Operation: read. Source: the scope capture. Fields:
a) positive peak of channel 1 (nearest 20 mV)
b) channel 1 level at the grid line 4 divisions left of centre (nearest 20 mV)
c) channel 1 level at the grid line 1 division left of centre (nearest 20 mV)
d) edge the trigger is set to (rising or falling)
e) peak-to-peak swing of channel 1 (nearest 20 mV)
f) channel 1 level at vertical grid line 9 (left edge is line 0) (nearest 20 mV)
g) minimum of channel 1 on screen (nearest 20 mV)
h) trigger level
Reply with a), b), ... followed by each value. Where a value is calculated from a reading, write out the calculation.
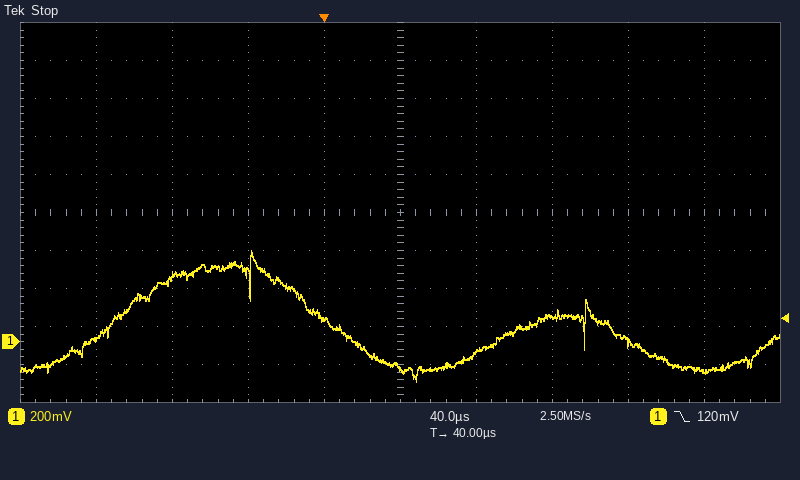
a) 480 mV
b) 20 mV
c) 120 mV
d) falling
e) 480 mV − (-200 mV) = 680 mV
f) -160 mV
g) -200 mV
h) 120 mV
